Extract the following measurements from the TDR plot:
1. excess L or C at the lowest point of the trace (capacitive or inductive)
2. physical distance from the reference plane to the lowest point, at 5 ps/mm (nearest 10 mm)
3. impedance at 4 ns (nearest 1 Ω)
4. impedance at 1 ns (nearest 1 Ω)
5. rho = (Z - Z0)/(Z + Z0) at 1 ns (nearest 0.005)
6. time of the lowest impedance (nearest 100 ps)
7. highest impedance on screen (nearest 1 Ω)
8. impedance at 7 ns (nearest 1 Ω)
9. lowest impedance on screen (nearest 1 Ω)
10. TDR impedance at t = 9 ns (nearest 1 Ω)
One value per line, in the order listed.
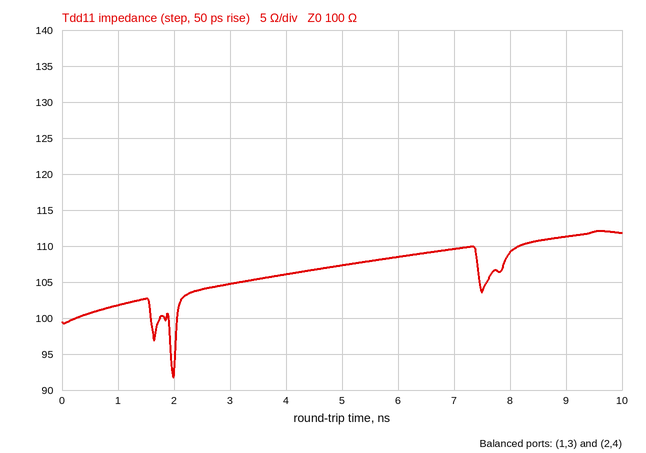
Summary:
capacitive
200 mm
106 Ω
102 Ω
+0.010
2.0 ns
112 Ω
110 Ω
92 Ω
111 Ω
